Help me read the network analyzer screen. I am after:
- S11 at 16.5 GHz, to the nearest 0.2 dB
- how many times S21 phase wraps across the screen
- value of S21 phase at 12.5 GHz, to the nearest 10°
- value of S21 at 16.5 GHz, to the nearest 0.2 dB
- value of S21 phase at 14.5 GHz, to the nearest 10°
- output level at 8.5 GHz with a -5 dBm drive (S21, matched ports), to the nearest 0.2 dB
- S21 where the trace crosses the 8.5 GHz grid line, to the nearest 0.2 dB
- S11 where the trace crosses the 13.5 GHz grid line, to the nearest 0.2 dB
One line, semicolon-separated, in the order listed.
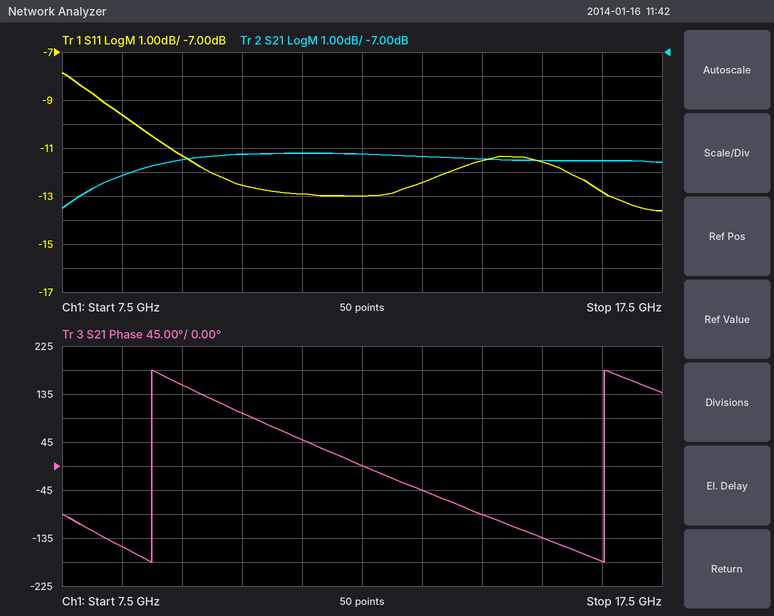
-12.8 dB; 2; 0°; -11.6 dB; -90°; -17.2 dBm; -12.2 dB; -12.4 dB
